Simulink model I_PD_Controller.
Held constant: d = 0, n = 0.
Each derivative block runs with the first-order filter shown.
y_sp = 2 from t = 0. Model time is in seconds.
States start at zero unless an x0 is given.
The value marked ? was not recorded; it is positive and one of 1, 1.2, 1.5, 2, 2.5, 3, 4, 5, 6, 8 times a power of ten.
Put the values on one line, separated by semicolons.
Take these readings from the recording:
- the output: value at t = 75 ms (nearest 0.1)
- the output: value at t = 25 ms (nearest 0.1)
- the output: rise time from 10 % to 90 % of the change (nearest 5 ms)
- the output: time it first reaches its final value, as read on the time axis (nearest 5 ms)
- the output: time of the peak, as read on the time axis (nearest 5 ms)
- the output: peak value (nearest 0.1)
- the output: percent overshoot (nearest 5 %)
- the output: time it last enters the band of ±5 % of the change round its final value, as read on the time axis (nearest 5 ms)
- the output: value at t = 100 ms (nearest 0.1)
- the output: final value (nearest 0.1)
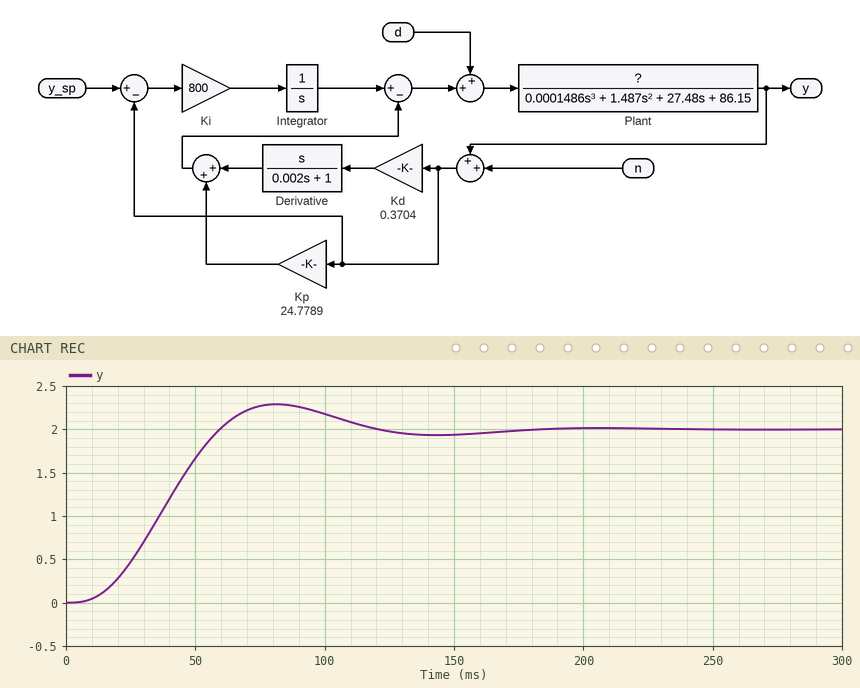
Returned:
2.3; 0.5; 35 ms; 60 ms; 80 ms; 2.3; 15 %; 110 ms; 2.2; 2.0
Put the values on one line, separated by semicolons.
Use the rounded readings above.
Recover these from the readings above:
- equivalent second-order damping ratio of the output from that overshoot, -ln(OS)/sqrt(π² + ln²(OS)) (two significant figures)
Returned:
0.52
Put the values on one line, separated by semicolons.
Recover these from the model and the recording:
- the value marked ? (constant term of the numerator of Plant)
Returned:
300
